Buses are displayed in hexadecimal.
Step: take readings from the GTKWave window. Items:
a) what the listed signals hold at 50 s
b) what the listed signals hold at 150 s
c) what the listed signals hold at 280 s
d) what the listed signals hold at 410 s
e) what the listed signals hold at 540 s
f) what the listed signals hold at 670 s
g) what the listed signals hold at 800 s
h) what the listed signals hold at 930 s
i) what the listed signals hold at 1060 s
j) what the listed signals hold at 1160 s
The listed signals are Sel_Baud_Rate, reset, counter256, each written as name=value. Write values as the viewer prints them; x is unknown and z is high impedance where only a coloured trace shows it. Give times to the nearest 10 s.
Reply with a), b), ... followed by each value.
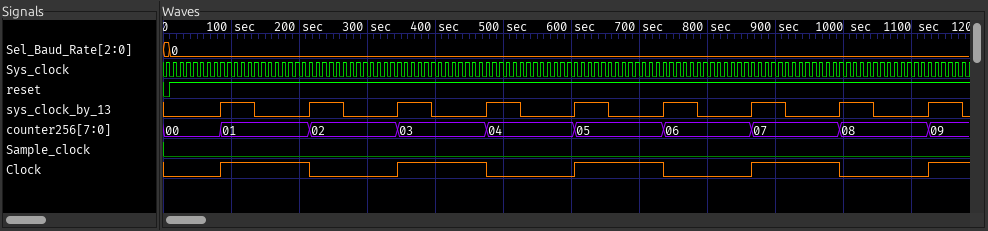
a) Sel_Baud_Rate=0, reset=1, counter256=00
b) Sel_Baud_Rate=0, reset=1, counter256=01
c) Sel_Baud_Rate=0, reset=1, counter256=02
d) Sel_Baud_Rate=0, reset=1, counter256=03
e) Sel_Baud_Rate=0, reset=1, counter256=04
f) Sel_Baud_Rate=0, reset=1, counter256=05
g) Sel_Baud_Rate=0, reset=1, counter256=06
h) Sel_Baud_Rate=0, reset=1, counter256=07
i) Sel_Baud_Rate=0, reset=1, counter256=08
j) Sel_Baud_Rate=0, reset=1, counter256=09
